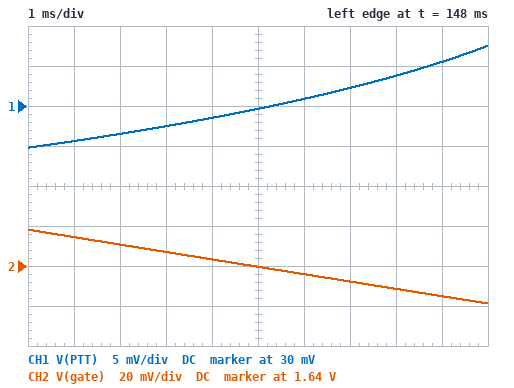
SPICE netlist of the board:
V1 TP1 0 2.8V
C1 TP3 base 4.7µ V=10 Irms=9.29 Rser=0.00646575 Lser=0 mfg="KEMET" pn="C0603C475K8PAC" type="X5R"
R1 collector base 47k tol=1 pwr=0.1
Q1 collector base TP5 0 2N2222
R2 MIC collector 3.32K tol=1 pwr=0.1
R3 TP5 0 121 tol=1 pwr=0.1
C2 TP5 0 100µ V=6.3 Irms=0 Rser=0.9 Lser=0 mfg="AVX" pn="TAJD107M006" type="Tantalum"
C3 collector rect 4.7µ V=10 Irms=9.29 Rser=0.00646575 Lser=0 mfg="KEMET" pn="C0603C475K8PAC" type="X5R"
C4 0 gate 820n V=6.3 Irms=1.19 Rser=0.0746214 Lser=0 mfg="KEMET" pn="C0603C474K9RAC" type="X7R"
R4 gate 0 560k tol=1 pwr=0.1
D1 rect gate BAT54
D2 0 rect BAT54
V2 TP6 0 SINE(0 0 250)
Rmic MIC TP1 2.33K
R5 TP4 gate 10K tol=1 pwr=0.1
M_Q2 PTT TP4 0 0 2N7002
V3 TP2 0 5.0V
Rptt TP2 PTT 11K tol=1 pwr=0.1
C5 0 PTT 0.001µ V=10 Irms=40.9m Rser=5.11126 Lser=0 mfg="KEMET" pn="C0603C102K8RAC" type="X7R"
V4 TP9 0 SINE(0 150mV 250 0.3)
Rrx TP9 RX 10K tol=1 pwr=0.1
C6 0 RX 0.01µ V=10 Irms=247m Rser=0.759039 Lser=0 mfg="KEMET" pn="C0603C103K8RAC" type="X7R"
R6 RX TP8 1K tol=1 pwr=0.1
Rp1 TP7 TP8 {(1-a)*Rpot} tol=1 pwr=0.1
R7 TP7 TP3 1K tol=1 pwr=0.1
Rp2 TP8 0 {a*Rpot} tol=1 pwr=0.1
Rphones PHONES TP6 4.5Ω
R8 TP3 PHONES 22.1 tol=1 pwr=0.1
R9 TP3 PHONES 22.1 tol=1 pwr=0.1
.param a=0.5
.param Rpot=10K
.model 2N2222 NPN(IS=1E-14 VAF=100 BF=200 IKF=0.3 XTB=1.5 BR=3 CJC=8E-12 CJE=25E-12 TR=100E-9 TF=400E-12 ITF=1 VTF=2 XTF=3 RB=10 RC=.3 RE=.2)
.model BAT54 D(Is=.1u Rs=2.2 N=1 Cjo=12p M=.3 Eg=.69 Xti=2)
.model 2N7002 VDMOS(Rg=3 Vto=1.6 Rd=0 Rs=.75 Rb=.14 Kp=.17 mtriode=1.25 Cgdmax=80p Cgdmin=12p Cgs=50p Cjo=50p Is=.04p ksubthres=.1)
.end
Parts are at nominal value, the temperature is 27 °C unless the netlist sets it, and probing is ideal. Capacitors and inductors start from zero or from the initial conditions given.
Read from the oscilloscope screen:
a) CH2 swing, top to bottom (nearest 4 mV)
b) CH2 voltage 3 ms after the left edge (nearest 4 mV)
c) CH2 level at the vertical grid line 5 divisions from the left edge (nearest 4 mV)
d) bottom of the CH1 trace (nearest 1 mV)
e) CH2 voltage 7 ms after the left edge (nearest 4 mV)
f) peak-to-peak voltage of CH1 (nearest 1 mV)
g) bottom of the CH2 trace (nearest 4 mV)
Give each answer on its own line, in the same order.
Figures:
36 mV
1.648 V
1.640 V
25 mV
1.632 V
13 mV
1.620 V
